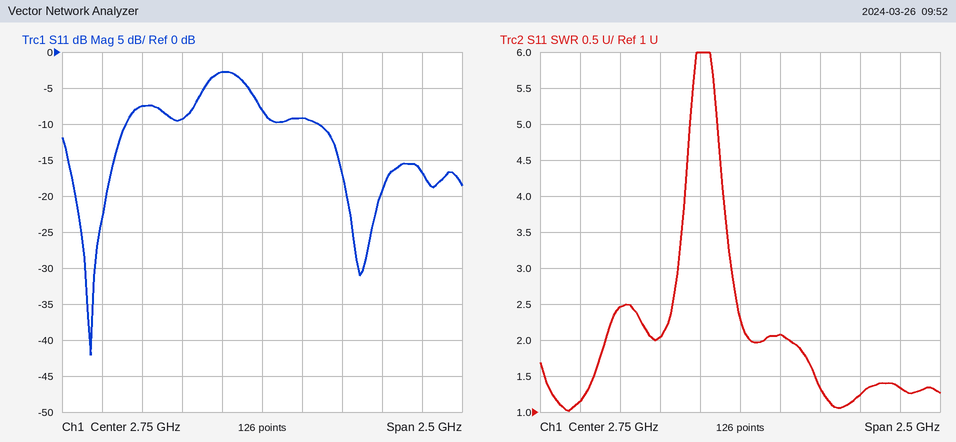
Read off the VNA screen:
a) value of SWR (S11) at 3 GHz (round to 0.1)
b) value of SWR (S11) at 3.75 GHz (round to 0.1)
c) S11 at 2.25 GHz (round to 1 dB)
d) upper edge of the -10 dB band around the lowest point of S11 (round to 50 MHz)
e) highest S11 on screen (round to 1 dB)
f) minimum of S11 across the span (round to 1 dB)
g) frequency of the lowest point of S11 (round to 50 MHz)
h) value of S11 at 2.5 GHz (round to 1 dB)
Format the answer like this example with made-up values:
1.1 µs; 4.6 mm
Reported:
2.1; 1.3; -9 dB; 1.90 GHz; -3 dB; -42 dB; 1.70 GHz; -3 dB
